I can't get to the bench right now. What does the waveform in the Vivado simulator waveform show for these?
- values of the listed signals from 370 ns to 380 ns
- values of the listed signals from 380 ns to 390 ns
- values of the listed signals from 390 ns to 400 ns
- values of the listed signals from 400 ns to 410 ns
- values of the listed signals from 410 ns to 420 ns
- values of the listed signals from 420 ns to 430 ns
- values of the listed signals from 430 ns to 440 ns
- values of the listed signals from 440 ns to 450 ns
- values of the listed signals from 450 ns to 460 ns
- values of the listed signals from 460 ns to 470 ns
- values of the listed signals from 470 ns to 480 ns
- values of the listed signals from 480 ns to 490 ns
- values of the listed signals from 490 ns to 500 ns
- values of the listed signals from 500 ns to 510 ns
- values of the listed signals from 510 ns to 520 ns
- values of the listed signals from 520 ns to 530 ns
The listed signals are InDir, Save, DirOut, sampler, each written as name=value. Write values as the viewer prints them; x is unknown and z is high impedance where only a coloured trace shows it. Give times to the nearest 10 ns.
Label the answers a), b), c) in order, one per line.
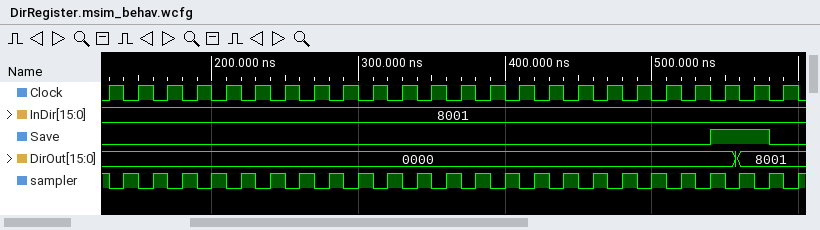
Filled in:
a) InDir=8001, Save=0, DirOut=0000, sampler=0
b) InDir=8001, Save=0, DirOut=0000, sampler=1
c) InDir=8001, Save=0, DirOut=0000, sampler=0
d) InDir=8001, Save=0, DirOut=0000, sampler=1
e) InDir=8001, Save=0, DirOut=0000, sampler=0
f) InDir=8001, Save=0, DirOut=0000, sampler=1
g) InDir=8001, Save=0, DirOut=0000, sampler=0
h) InDir=8001, Save=0, DirOut=0000, sampler=1
i) InDir=8001, Save=0, DirOut=0000, sampler=0
j) InDir=8001, Save=0, DirOut=0000, sampler=1
k) InDir=8001, Save=0, DirOut=0000, sampler=0
l) InDir=8001, Save=0, DirOut=0000, sampler=1
m) InDir=8001, Save=0, DirOut=0000, sampler=0
n) InDir=8001, Save=0, DirOut=0000, sampler=1
o) InDir=8001, Save=0, DirOut=0000, sampler=0
p) InDir=8001, Save=0, DirOut=0000, sampler=1
